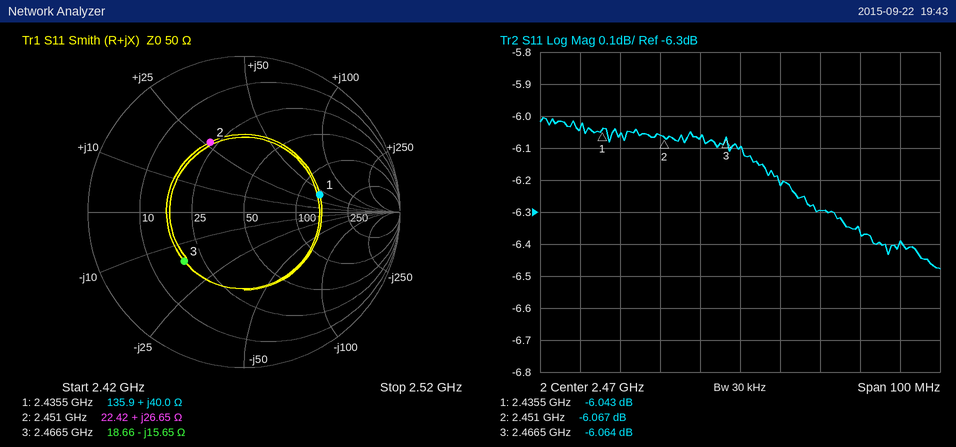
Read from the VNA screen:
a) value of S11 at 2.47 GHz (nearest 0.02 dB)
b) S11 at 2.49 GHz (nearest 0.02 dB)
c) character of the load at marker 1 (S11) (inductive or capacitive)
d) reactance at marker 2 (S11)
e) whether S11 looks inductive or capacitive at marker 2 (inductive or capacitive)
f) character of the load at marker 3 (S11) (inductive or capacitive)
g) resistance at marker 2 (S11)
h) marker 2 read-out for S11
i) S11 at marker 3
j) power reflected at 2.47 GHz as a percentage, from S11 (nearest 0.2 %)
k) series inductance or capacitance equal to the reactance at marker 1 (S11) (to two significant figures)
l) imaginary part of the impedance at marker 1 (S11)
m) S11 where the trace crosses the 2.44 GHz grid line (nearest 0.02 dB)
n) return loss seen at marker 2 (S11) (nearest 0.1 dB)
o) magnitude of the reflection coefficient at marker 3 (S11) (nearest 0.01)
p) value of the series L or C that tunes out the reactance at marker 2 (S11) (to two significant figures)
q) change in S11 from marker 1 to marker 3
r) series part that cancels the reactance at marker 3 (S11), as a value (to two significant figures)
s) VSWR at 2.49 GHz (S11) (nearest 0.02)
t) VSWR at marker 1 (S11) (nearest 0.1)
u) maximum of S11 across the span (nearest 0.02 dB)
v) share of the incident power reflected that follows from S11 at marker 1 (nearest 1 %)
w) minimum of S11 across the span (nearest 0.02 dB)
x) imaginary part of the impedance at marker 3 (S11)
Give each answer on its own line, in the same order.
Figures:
-6.10 dB
-6.30 dB
inductive
+26.65 Ω
inductive
capacitive
22.42 Ω
-6.067 dB
-6.064 dB
24.6 %
2.6 nH
+40.0 Ω
-6.06 dB
6.1 dB
0.50
2.4 pF
-0.021 dB
1.0 nH
2.88
3.0
-6.00 dB
25 %
-6.48 dB
-15.65 Ω
